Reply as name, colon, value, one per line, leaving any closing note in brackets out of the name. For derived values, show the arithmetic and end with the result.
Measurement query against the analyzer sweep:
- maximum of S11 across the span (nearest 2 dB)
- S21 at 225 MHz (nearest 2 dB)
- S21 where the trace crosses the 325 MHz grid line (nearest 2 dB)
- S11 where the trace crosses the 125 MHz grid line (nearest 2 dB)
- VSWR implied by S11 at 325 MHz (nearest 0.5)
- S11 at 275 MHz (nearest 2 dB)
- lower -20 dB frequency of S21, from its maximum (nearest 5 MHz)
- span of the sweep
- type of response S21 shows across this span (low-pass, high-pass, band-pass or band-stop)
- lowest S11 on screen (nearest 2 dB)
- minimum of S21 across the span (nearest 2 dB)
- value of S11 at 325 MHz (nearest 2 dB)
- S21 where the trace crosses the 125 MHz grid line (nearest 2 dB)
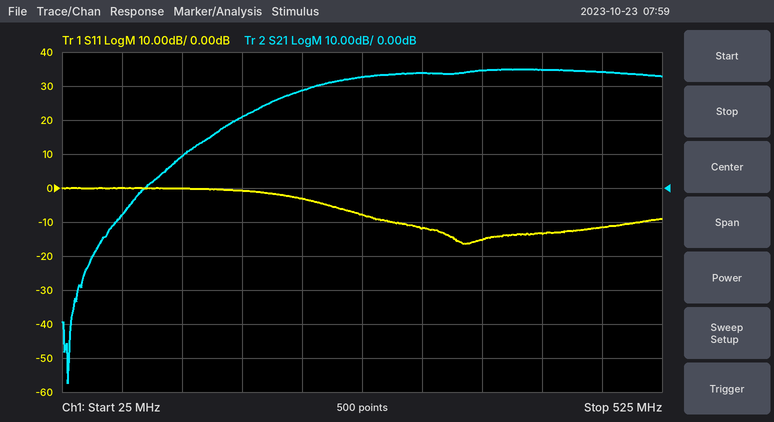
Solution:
maximum of S11 across the span: 0 dB
S21 at 225 MHz: 28 dB
S21 where the trace crosses the 325 MHz grid line: 34 dB
S11 where the trace crosses the 125 MHz grid line: 0 dB
VSWR implied by S11 at 325 MHz: |Γ| = 10^(-12/20) = 0.2512; VSWR = (1 + 0.2512)/(1 − 0.2512) ≈ 1.67, so 1.5 to the nearest 0.5
S11 at 275 MHz: -8 dB
lower -20 dB frequency of S21, from its maximum: 150 MHz
span of the sweep: 500 MHz
type of response S21 shows across this span: high-pass
lowest S11 on screen: -16 dB
minimum of S21 across the span: -58 dB
value of S11 at 325 MHz: -12 dB
S21 where the trace crosses the 125 MHz grid line: 10 dB
